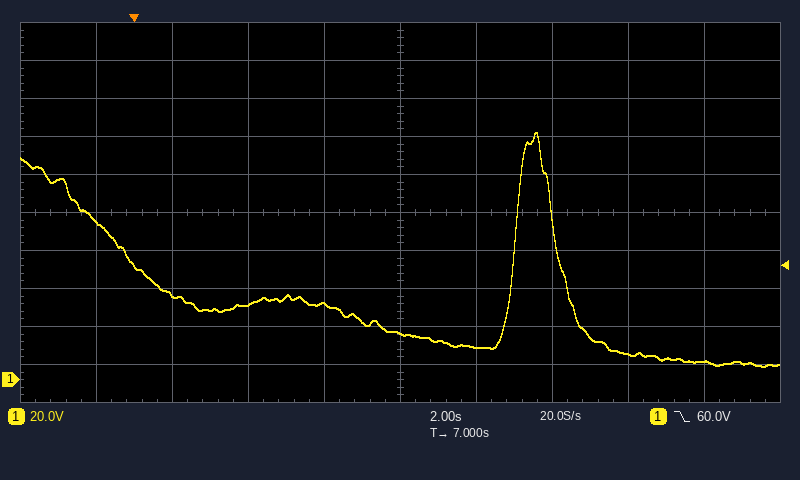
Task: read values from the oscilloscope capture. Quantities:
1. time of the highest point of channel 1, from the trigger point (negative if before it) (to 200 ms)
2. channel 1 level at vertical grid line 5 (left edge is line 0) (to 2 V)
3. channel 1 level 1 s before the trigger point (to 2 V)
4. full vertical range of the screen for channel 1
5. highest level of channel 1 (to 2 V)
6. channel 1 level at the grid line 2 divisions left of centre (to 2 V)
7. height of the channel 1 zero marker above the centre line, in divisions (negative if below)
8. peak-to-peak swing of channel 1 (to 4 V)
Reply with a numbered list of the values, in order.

1. +10.6 s
2. 24 V
3. 84 V
4. 200 V
5. 130 V
6. 40 V
7. -4.4 div
8. 124 V
